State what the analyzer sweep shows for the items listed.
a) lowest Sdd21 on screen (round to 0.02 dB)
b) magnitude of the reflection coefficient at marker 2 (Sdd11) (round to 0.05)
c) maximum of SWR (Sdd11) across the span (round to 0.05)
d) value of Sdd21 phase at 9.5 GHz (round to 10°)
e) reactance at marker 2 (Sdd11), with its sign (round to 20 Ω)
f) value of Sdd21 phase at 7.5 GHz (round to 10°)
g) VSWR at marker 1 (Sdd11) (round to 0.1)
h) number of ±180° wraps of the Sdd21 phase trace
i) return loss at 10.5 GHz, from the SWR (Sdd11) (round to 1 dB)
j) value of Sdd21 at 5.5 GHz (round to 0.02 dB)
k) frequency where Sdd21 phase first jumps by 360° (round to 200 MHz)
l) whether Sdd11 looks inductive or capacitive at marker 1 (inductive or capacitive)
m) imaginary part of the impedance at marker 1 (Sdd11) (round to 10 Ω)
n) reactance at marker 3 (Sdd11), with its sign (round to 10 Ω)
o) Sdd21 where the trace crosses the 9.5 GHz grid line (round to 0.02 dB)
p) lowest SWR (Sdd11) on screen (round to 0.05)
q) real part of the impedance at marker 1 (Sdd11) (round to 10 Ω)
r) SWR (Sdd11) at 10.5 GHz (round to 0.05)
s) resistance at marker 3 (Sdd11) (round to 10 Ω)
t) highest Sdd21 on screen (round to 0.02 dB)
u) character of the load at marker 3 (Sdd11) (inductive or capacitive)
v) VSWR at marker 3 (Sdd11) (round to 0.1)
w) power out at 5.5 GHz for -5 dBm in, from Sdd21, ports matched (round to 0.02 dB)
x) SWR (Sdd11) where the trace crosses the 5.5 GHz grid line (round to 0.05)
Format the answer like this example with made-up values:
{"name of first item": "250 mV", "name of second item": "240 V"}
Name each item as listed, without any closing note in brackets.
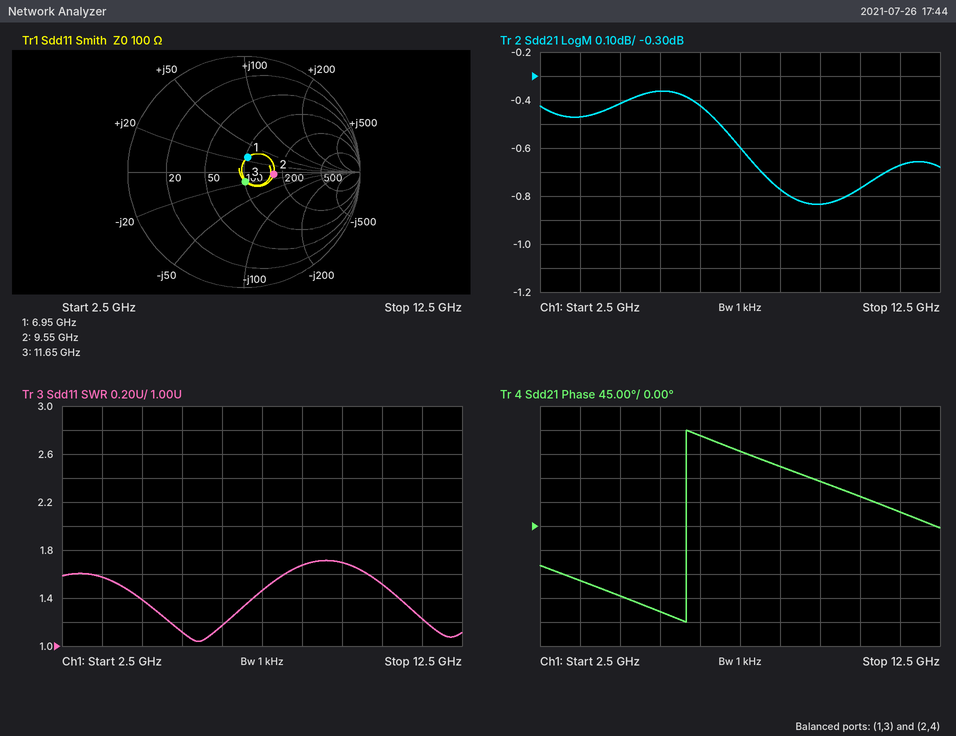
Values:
{"lowest Sdd21 on screen": "-0.84 dB", "magnitude of the reflection coefficient at marker 2 (Sdd11)": "0.25", "maximum of SWR (Sdd11) across the span": "1.70", "value of Sdd21 phase at 9.5 GHz": "80°", "reactance at marker 2 (Sdd11), with its sign": "0 Ω", "value of Sdd21 phase at 7.5 GHz": "140°", "VSWR at marker 1 (Sdd11)": "1.3", "number of ±180° wraps of the Sdd21 phase trace": "1", "return loss at 10.5 GHz, from the SWR (Sdd11)": "14 dB", "value of Sdd21 at 5.5 GHz": "-0.36 dB", "frequency where Sdd21 phase first jumps by 360°": "6.2 GHz", "whether Sdd11 looks inductive or capacitive at marker 1": "inductive", "imaginary part of the impedance at marker 1 (Sdd11)": "+30 Ω", "reactance at marker 3 (Sdd11), with its sign": "-20 Ω", "Sdd21 where the trace crosses the 9.5 GHz grid line": "-0.84 dB", "lowest SWR (Sdd11) on screen": "1.05", "real part of the impedance at marker 1 (Sdd11)": "100 Ω", "SWR (Sdd11) at 10.5 GHz": "1.50", "resistance at marker 3 (Sdd11)": "100 Ω", "highest Sdd21 on screen": "-0.36 dB", "character of the load at marker 3 (Sdd11)": "capacitive", "VSWR at marker 3 (Sdd11)": "1.2", "power out at 5.5 GHz for -5 dBm in, from Sdd21, ports matched": "-5.36 dBm", "SWR (Sdd11) where the trace crosses the 5.5 GHz grid line": "1.10"}
